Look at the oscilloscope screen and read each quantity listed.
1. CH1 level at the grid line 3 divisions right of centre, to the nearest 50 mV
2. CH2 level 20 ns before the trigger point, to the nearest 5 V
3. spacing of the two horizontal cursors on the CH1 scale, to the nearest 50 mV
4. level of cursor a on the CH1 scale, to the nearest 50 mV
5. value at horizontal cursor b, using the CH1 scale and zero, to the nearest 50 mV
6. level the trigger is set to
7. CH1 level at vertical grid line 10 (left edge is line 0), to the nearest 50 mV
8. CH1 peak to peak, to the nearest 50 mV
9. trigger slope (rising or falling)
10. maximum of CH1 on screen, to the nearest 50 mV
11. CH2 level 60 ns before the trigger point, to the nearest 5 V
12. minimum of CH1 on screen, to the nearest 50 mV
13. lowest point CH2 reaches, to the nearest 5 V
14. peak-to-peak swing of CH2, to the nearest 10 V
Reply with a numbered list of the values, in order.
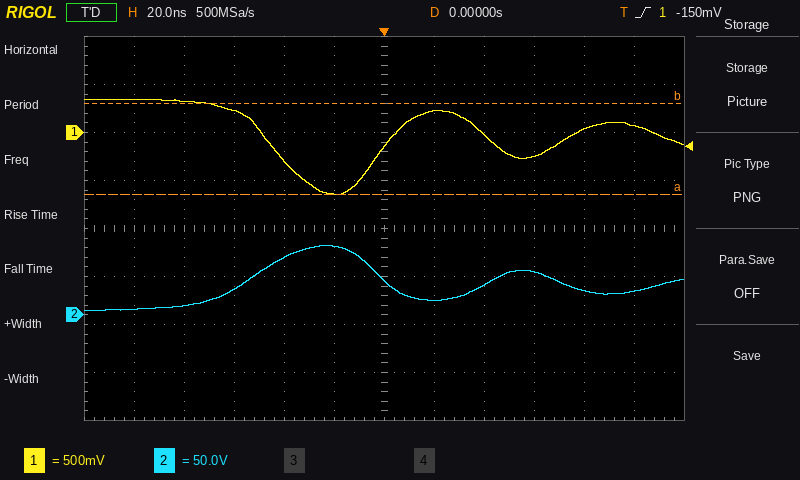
1. -250 mV
2. 70 V
3. 950 mV
4. -650 mV
5. 300 mV
6. -150 mV
7. 50 mV
8. 1.00 V
9. rising
10. 350 mV
11. 25 V
12. -650 mV
13. 5 V
14. 70 V
